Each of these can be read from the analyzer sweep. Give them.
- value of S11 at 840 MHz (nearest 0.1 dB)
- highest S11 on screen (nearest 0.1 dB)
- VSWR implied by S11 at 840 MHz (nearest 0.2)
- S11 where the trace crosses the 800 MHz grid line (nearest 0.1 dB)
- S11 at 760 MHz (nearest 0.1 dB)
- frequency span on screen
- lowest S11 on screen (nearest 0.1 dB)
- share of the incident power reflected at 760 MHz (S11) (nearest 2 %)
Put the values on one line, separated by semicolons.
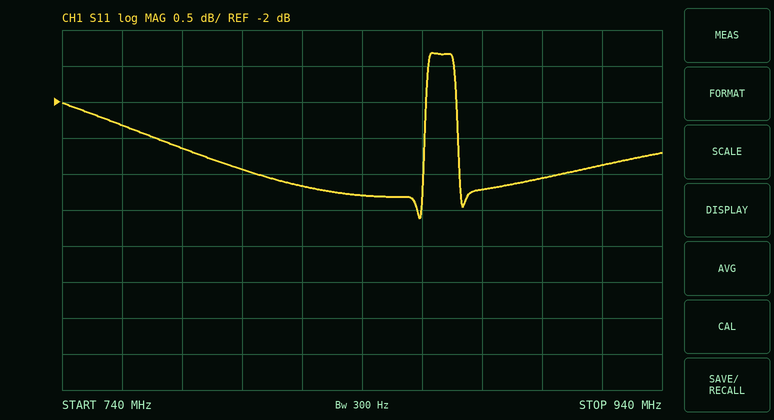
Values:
-3.3 dB; -1.3 dB; 5.4; -2.9 dB; -2.3 dB; 200 MHz; -3.6 dB; 58 %
